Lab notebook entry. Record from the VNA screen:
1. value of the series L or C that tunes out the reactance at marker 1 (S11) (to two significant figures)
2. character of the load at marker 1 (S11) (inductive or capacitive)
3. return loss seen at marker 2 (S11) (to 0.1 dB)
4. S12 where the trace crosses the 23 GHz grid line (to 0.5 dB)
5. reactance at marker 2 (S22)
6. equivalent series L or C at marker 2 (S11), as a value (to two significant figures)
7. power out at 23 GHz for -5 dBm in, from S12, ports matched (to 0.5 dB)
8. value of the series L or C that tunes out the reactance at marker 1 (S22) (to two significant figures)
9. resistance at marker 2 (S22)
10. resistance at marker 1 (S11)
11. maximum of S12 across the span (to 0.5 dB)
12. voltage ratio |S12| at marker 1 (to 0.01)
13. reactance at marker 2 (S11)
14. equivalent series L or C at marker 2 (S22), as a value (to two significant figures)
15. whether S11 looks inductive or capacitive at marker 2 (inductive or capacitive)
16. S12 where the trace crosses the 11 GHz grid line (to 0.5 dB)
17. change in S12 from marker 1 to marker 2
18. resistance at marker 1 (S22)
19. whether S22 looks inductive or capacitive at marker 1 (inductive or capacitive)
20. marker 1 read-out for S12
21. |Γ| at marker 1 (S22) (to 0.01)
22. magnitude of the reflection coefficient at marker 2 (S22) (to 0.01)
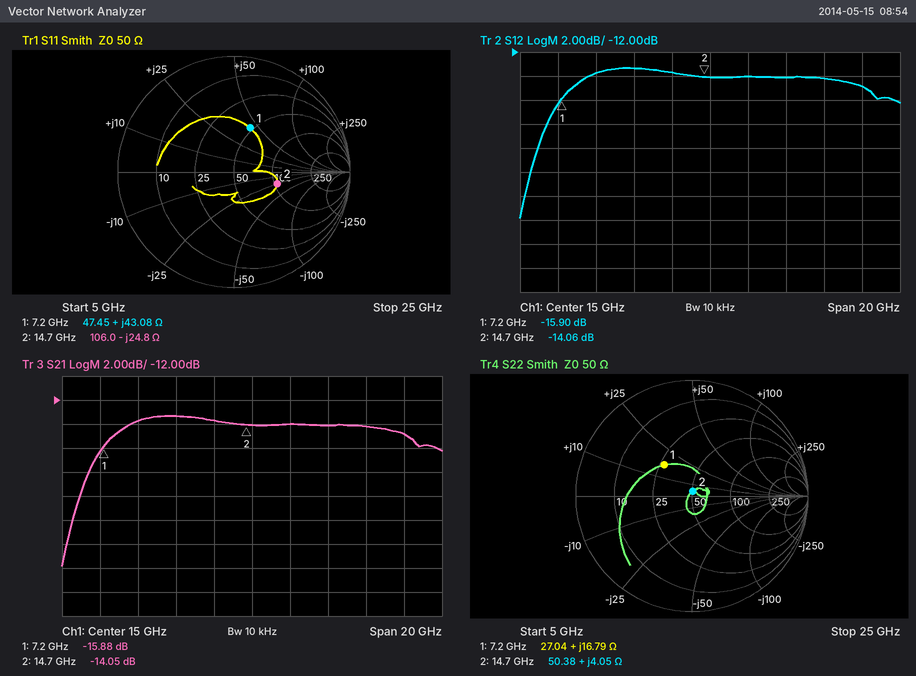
510 fF
inductive
8.2 dB
-15.0 dB
+4.05 Ω
440 fF
-20.0 dBm
1.3 pF
50.38 Ω
47.45 Ω
-13.5 dB
0.16
-24.8 Ω
44 pH
capacitive
-13.5 dB
1.84 dB
27.04 Ω
inductive
-15.90 dB
0.36
0.04
